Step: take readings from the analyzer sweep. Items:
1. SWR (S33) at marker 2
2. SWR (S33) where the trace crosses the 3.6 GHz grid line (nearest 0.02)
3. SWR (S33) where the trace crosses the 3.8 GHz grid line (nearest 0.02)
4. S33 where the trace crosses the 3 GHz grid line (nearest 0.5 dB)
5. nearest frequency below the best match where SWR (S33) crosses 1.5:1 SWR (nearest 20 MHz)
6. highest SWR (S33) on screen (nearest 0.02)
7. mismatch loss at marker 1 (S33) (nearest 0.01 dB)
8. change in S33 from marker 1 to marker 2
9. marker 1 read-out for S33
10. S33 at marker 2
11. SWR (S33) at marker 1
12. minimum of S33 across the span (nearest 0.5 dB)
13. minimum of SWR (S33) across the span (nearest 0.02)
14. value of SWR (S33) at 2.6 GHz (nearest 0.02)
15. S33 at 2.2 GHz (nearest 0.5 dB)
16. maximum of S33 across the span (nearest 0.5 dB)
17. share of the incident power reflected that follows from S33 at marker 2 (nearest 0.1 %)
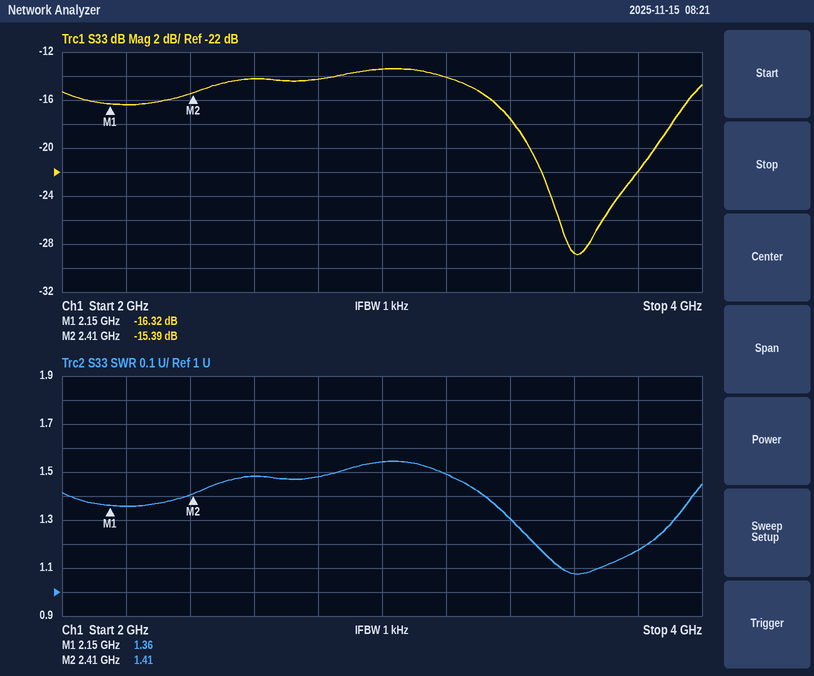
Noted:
1.41
1.08
1.18
-13.5 dB
3.18 GHz
1.54
0.10 dB
0.93 dB
-16.32 dB
-15.39 dB
1.36
-29.0 dB
1.08
1.48
-16.5 dB
-13.5 dB
2.9 %
